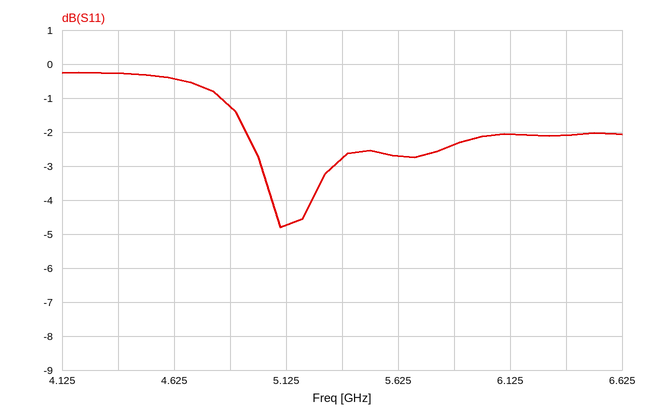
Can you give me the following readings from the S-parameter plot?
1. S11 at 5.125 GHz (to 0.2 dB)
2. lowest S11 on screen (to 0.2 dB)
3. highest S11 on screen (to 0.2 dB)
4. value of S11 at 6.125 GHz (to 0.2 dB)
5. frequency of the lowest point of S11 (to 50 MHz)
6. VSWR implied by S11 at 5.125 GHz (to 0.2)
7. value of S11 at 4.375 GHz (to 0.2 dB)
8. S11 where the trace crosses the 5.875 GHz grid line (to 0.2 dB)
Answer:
-4.8 dB
-4.8 dB
-0.2 dB
-2.0 dB
5.10 GHz
3.8
-0.2 dB
-2.4 dB
